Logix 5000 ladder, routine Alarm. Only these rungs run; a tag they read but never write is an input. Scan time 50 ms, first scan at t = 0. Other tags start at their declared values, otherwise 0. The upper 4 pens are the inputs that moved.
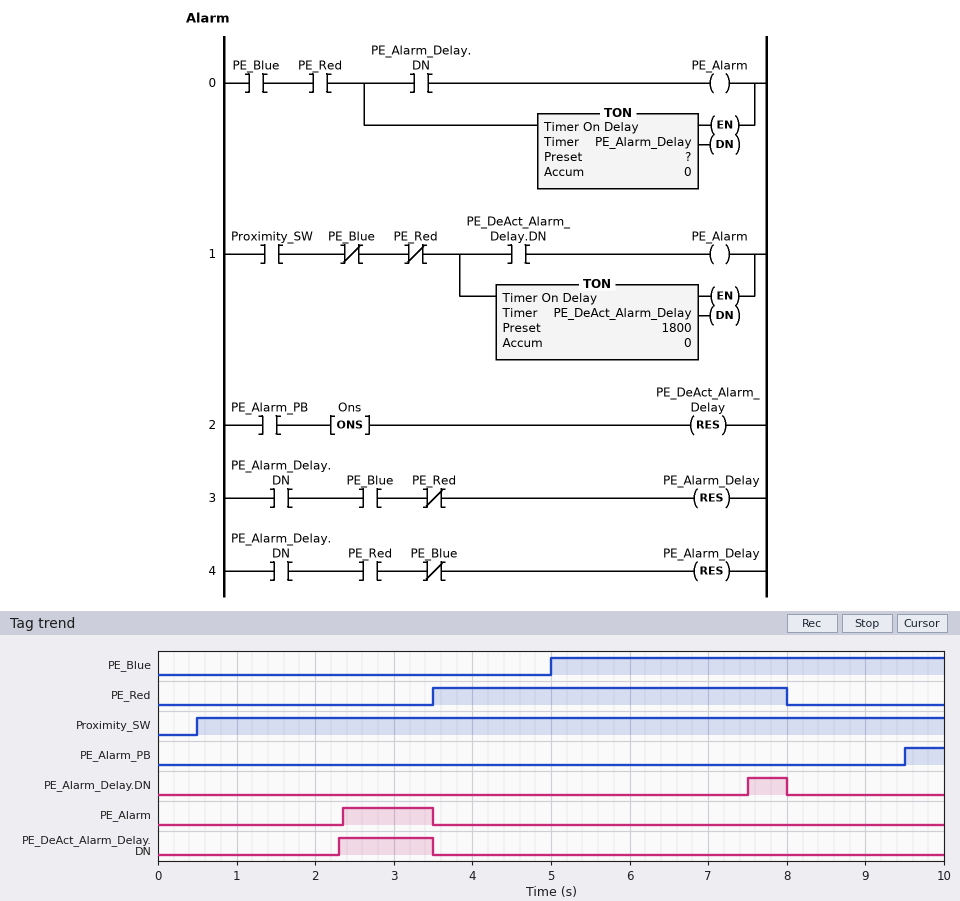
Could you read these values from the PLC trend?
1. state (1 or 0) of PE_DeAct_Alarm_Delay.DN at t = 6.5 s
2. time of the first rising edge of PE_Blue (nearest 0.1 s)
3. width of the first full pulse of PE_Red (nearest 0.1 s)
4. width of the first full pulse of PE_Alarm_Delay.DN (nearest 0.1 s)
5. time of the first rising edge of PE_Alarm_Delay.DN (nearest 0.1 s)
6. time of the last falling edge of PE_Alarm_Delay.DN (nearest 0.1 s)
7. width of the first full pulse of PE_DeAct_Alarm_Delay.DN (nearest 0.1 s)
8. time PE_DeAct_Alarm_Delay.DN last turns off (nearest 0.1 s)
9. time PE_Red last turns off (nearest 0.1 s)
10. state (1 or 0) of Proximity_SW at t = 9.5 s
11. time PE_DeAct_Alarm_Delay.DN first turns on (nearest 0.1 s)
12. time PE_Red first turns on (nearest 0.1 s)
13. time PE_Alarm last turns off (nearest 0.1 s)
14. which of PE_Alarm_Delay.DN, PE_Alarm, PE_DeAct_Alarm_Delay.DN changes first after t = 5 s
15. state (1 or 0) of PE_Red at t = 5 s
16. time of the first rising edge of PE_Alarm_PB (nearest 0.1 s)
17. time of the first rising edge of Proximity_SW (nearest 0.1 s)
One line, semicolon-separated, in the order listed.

0; 5.0 s; 4.5 s; 0.5 s; 7.5 s; 8.0 s; 1.2 s; 3.5 s; 8.0 s; 1; 2.3 s; 3.5 s; 3.5 s; PE_Alarm_Delay.DN; 1; 9.5 s; 0.5 s
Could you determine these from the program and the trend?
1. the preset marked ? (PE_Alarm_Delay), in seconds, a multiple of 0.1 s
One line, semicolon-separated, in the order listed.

2.5 s
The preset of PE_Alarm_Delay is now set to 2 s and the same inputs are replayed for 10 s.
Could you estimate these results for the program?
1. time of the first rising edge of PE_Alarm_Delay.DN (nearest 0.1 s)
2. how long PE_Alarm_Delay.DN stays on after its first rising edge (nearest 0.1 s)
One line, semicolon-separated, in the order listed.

7.0 s; 1.0 s
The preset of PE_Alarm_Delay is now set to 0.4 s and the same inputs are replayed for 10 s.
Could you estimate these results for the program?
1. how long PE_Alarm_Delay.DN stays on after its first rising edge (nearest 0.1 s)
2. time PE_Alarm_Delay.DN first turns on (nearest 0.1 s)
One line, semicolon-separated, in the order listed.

2.6 s; 5.4 s
